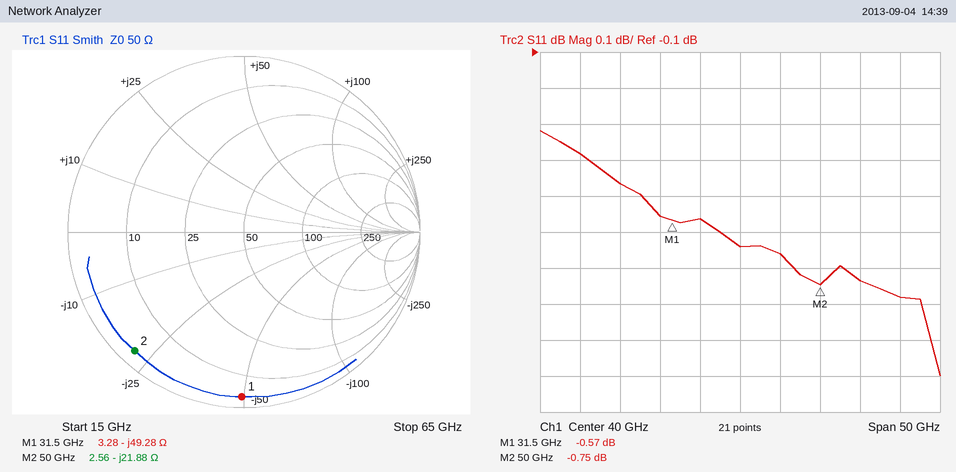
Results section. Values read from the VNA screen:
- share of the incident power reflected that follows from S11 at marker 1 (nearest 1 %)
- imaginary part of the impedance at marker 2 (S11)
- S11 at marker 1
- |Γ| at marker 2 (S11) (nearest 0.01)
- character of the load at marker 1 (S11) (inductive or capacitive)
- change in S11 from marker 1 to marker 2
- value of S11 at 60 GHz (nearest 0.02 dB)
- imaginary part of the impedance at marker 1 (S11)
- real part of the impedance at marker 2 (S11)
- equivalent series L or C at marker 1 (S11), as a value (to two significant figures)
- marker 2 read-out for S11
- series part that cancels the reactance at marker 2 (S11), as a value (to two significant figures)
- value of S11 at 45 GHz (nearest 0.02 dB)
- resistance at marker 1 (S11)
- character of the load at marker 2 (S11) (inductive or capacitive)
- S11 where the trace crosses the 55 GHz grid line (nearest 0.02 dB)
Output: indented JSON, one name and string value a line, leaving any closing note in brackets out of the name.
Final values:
{
  "share of the incident power reflected that follows from S11 at marker 1": "88 %",
  "imaginary part of the impedance at marker 2": "-21.88 Ω",
  "S11 at marker 1": "-0.57 dB",
  "|Γ| at marker 2 (S11)": "0.92",
  "character of the load at marker 1 (S11)": "capacitive",
  "change in S11 from marker 1 to marker 2": "-0.18 dB",
  "value of S11 at 60 GHz": "-0.78 dB",
  "imaginary part of the impedance at marker 1": "-49.28 Ω",
  "real part of the impedance at marker 2": "2.56 Ω",
  "equivalent series L or C at marker 1 (S11), as a value": "100 fF",
  "marker 2 read-out for S11": "-0.75 dB",
  "series part that cancels the reactance at marker 2 (S11), as a value": "70 pH",
  "value of S11 at 45 GHz": "-0.66 dB",
  "resistance at marker 1": "3.28 Ω",
  "character of the load at marker 2 (S11)": "capacitive",
  "S11 where the trace crosses the 55 GHz grid line": "-0.74 dB"
}
